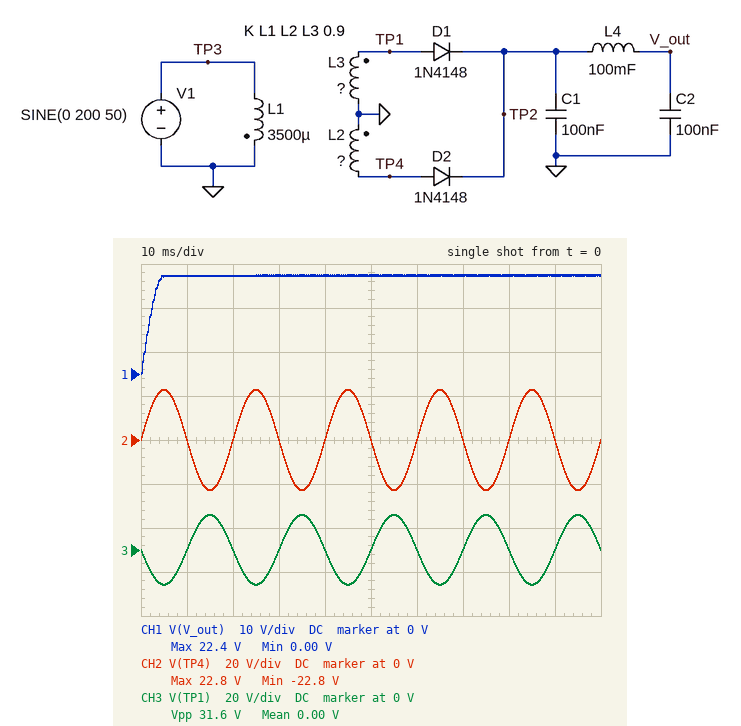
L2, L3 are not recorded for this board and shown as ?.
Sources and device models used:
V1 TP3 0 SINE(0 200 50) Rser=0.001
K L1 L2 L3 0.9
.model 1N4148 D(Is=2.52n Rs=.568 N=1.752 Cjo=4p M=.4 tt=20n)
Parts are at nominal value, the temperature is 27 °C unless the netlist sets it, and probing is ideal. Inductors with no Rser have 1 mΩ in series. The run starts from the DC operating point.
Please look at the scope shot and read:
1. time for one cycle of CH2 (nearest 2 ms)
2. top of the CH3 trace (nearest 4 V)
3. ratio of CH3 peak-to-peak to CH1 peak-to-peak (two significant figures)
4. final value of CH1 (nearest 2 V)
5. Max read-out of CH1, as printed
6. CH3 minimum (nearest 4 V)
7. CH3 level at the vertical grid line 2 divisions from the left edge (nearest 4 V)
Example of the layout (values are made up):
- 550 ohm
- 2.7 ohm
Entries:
- 20 ms
- 16 V
- 1.4
- 22 V
- 22.4 V
- -16 V
- 0 V
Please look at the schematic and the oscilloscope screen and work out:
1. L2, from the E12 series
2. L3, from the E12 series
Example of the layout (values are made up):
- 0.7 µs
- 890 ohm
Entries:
- 56 µH
- 27 µH
